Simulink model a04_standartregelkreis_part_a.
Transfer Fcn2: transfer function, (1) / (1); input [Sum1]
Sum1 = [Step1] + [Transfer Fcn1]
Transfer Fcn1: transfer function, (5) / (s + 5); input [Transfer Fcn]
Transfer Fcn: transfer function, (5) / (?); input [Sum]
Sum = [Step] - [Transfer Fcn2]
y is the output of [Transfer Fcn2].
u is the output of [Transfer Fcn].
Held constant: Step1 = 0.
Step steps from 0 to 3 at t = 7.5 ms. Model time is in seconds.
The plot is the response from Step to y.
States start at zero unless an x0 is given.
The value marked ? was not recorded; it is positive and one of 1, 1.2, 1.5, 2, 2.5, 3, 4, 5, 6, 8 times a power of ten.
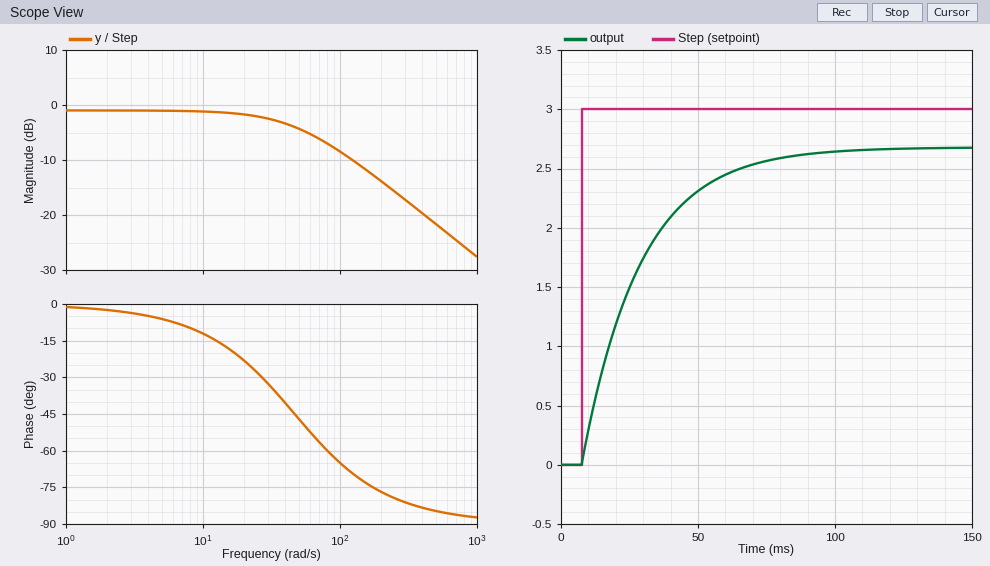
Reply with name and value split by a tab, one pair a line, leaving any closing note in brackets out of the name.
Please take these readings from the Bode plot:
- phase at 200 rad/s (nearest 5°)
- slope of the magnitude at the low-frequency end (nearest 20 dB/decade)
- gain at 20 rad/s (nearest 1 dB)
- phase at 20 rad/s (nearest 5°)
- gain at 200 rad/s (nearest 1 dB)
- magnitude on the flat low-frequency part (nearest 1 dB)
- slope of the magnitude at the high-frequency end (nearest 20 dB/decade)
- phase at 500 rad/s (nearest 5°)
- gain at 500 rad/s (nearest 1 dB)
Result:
phase at 200 rad/s	-75°
slope of the magnitude at the low-frequency end	0 dB/decade
gain at 20 rad/s	-2 dB
phase at 20 rad/s	-25°
gain at 200 rad/s	-14 dB
magnitude on the flat low-frequency part	-1 dB
slope of the magnitude at the high-frequency end	-20 dB/decade
phase at 500 rad/s	-85°
gain at 500 rad/s	-22 dB
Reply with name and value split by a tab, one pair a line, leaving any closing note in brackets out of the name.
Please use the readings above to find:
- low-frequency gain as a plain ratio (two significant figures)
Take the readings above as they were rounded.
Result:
low-frequency gain as a plain ratio	0.89
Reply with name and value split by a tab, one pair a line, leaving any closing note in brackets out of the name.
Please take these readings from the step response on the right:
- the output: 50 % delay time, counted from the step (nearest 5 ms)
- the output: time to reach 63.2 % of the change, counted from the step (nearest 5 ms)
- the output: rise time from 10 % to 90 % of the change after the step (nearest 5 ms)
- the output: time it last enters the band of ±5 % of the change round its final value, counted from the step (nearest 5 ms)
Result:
the output: 50 % delay time, counted from the step	15 ms
the output: time to reach 63.2 % of the change, counted from the step	20 ms
the output: rise time from 10 % to 90 % of the change after the step	45 ms
the output: time it last enters the band of ±5 % of the change round its final value, counted from the step	65 ms
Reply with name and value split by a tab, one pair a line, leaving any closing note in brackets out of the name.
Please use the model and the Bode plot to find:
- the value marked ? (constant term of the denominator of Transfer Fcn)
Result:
the value marked ?	0.6
